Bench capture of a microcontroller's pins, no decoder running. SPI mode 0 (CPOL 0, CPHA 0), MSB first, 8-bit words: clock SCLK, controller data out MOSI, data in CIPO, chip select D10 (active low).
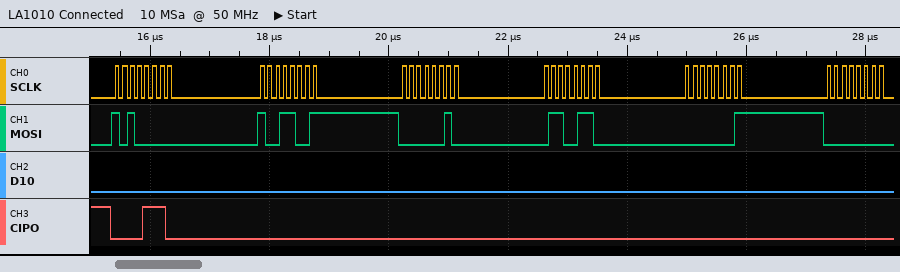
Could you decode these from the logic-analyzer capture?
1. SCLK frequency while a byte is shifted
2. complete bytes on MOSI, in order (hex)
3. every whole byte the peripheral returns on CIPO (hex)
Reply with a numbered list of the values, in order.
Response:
1. 8 MHz
2. 0xA0 0x99 0x02 0x66 0x01 0x00
3. 0x0E 0x00 0x00 0x00 0x00 0x00
